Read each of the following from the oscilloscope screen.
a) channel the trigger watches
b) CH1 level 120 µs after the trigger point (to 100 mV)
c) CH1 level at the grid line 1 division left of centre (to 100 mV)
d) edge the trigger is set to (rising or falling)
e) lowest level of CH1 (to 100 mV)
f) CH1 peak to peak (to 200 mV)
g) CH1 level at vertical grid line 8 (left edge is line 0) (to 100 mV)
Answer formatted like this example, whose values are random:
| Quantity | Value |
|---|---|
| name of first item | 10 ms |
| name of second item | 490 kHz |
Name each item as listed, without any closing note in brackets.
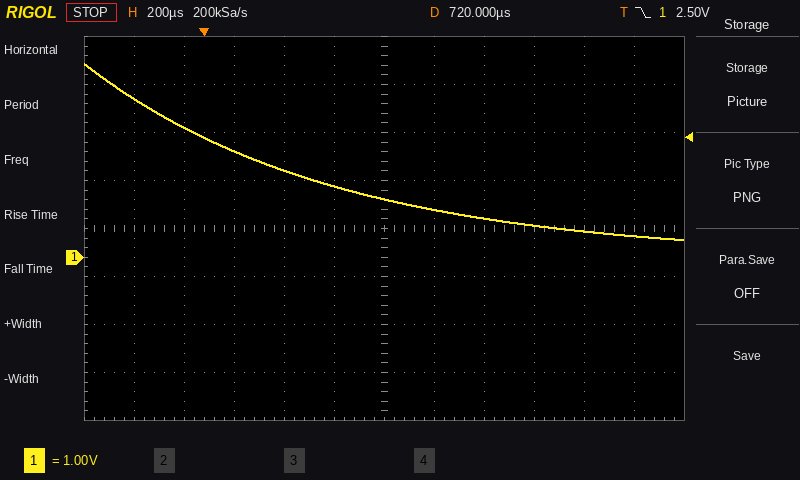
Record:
| Quantity | Value |
|---|---|
| channel the trigger watches | CH1 |
| CH1 level 120 µs after the trigger point | 2.2 V |
| CH1 level at the grid line 1 division left of centre | 1.5 V |
| edge the trigger is set to | falling |
| lowest level of CH1 | 400 mV |
| CH1 peak to peak | 3.6 V |
| CH1 level at vertical grid line 8 (left edge is line 0) | 800 mV |
